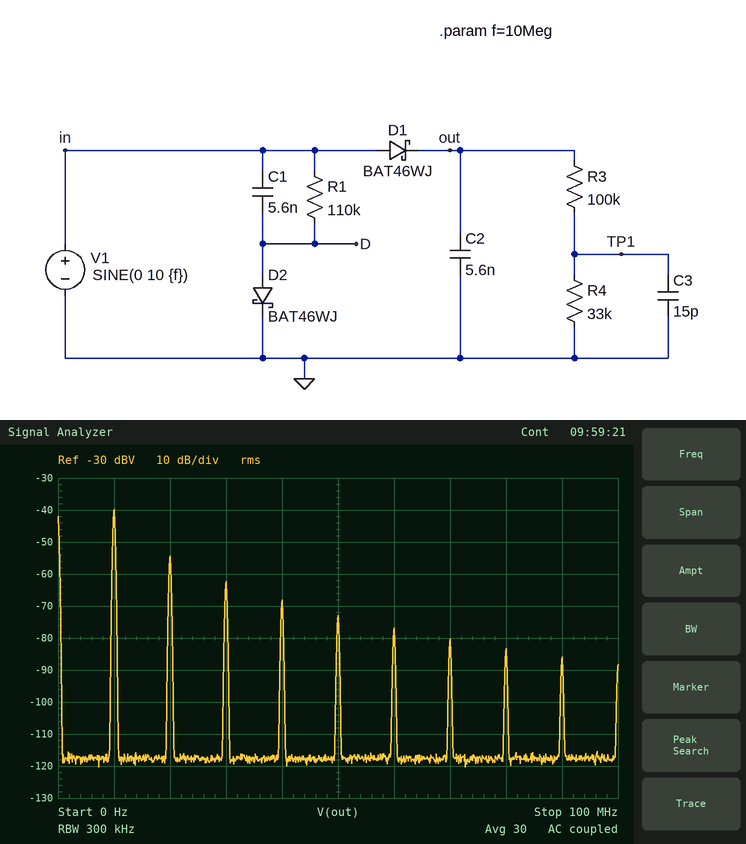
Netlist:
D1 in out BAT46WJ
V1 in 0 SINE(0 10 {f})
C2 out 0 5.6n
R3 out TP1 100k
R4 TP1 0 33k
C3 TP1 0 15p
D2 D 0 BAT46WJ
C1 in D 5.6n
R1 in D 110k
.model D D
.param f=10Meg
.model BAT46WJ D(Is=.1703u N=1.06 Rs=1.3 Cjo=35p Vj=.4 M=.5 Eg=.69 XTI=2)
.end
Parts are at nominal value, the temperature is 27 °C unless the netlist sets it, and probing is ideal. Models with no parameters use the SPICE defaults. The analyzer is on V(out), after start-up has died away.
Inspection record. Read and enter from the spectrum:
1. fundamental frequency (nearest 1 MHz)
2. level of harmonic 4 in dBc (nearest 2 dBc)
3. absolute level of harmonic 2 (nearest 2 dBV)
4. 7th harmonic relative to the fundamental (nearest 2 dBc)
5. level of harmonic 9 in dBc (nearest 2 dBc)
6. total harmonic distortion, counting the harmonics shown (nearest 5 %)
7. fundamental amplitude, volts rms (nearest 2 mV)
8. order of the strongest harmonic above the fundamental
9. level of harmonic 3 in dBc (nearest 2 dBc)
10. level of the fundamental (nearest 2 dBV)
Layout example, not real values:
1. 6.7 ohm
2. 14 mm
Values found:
1. 10 MHz
2. -28 dBc
3. -54 dBV
4. -40 dBc
5. -46 dBc
6. 20 %
7. 10 mV
8. 2
9. -22 dBc
10. -40 dBV
